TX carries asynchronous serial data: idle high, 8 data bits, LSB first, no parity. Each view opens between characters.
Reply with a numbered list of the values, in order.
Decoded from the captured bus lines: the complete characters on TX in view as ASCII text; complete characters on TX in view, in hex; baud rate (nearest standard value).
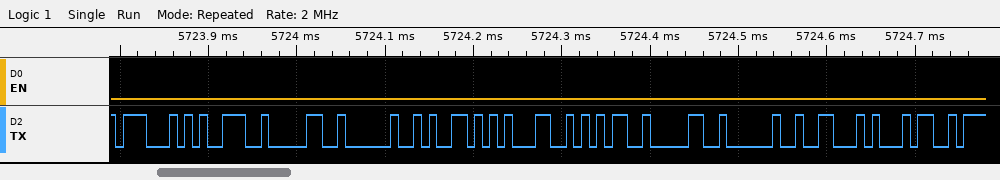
1. "G90 Y150 F4"
2. 47, 39, 30, 20, 59, 31, 35, 30, 20, 46, 34
3. 115200 baud
